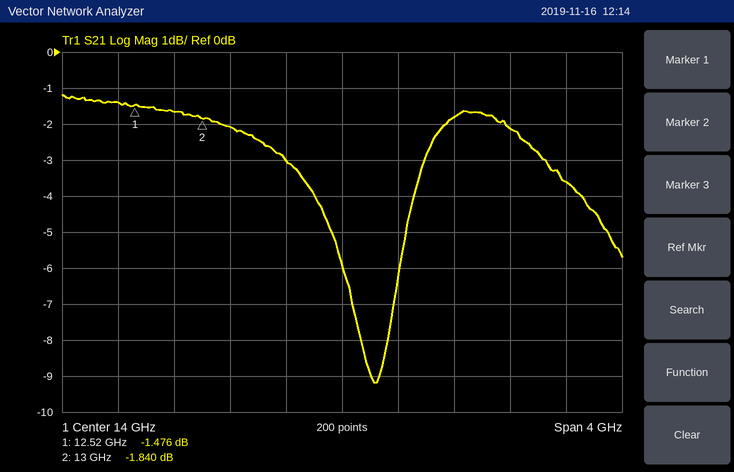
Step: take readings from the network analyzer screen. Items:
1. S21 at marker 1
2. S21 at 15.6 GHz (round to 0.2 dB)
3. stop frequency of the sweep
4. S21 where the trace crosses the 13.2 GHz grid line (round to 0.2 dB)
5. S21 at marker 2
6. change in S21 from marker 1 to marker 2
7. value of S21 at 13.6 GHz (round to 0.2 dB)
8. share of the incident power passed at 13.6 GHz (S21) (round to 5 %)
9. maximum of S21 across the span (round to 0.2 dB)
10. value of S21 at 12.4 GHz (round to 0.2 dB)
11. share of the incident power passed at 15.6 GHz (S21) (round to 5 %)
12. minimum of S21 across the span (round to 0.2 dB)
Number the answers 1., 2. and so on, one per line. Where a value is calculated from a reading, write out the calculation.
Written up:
1. -1.476 dB
2. -3.6 dB
3. 16 GHz
4. -2.0 dB
5. -1.840 dB
6. -1.84 − (-1.476) = -0.364 dB
7. -3.0 dB
8. 10^(-3/10) ≈ 50 %
9. -1.2 dB
10. -1.4 dB
11. 10^(-3.6/10) ≈ 43.7 %, so 45 % to the nearest 5 %
12. -9.2 dB
